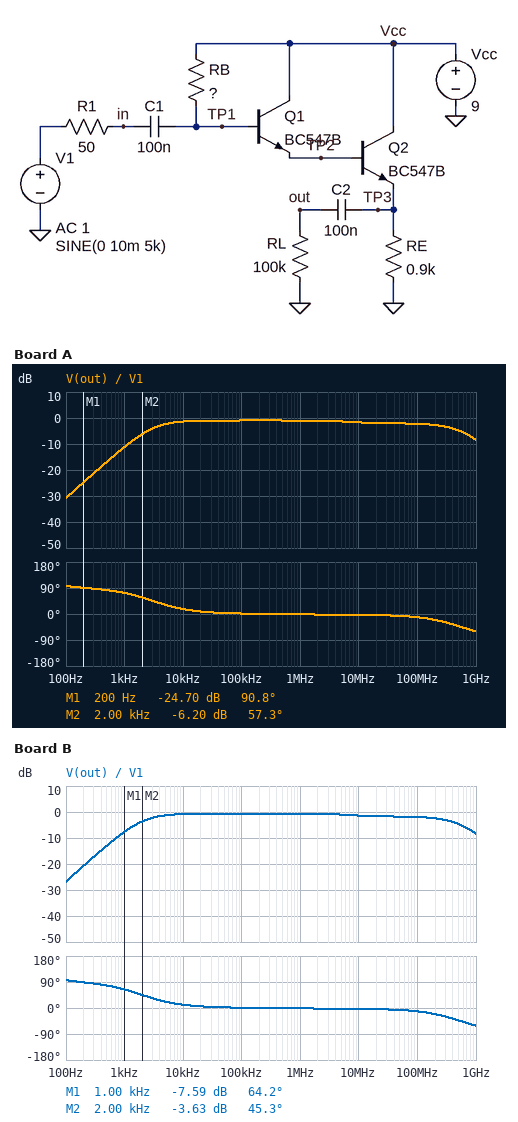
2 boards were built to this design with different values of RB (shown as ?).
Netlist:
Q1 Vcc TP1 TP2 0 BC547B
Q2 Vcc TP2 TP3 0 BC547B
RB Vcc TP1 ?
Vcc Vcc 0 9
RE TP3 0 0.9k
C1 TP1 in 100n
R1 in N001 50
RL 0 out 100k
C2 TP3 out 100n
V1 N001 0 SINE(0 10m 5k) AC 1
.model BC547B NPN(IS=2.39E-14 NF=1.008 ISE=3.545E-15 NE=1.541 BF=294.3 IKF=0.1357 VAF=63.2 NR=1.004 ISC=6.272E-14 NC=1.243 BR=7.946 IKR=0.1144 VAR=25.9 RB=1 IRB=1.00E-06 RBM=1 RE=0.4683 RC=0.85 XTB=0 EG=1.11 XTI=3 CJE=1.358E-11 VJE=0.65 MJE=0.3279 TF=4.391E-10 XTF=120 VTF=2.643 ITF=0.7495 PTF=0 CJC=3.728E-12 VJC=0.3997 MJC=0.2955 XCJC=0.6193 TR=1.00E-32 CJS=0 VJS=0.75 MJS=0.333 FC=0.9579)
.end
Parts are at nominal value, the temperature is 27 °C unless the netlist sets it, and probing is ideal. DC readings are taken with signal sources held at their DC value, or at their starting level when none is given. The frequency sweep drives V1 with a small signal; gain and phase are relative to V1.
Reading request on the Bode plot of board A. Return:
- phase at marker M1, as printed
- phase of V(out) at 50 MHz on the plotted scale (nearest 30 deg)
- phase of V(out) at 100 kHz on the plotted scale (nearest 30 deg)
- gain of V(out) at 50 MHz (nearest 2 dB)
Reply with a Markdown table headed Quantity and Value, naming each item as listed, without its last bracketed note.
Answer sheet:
| Quantity | Value |
|---|---|
| phase at marker M1, as printed | 90.8 deg |
| phase of V(out) at 50 MHz on the plotted scale | 0 deg |
| phase of V(out) at 100 kHz on the plotted scale | 0 deg |
| gain of V(out) at 50 MHz | -2 dB |
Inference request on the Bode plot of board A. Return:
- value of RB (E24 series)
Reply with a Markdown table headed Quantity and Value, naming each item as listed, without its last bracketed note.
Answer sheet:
| Quantity | Value |
|---|---|
| value of RB | 470 Ω |
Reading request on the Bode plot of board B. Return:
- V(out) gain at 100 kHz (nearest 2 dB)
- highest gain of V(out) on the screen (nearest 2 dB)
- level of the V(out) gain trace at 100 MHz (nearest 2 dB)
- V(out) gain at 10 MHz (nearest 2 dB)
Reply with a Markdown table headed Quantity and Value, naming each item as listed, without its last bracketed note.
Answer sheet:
| Quantity | Value |
|---|---|
| V(out) gain at 100 kHz | 0 dB |
| highest gain of V(out) on the screen | 0 dB |
| level of the V(out) gain trace at 100 MHz | -2 dB |
| V(out) gain at 10 MHz | -2 dB |
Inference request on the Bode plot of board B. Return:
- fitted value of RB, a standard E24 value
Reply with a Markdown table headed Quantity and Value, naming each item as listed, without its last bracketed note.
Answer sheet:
| Quantity | Value |
|---|---|
| fitted value of RB, a standard E24 value | 750 Ω |
